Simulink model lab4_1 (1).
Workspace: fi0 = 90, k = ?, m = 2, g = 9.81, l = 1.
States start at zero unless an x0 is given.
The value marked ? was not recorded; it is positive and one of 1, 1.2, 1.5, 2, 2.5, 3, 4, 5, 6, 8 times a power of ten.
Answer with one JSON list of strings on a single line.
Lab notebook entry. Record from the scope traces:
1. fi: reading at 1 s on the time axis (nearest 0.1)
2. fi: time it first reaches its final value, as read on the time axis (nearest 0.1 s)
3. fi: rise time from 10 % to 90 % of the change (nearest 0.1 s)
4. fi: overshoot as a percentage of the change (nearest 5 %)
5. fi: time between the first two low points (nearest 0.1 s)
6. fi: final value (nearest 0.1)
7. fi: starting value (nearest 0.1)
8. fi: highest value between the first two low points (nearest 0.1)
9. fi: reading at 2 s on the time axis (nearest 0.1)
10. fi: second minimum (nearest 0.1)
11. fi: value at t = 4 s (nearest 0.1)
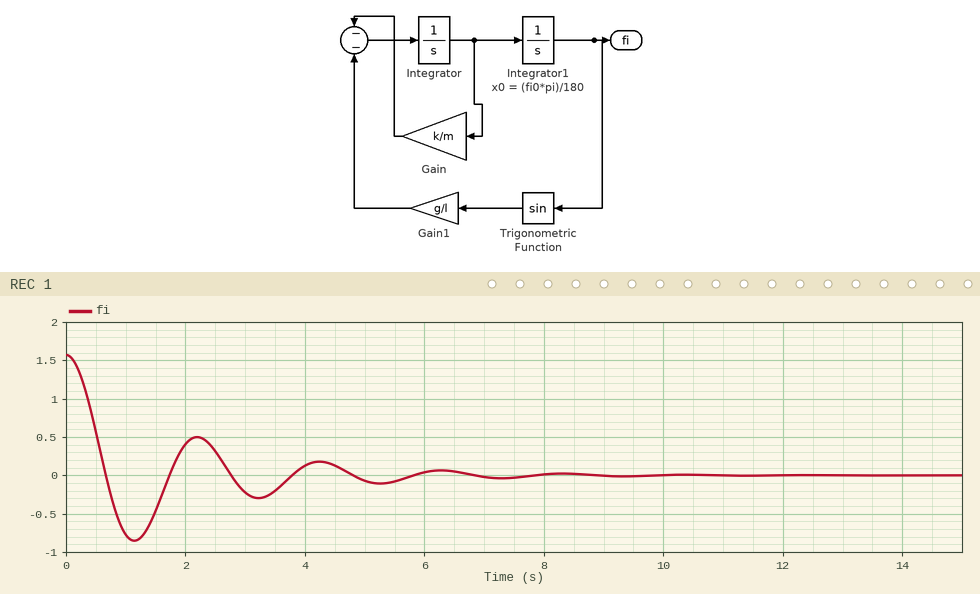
["-0.8", "0.7 s", "0.4 s", "55 %", "2.1 s", "0.0", "1.6", "0.5", "0.4", "-0.3", "0.1"]
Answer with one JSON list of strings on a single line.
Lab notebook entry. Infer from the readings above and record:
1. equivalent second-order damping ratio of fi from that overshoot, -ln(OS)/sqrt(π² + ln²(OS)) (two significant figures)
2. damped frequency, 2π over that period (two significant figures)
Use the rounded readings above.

["0.19", "3.0 rad/s"]
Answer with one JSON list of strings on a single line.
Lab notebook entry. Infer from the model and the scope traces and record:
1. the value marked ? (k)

["2"]
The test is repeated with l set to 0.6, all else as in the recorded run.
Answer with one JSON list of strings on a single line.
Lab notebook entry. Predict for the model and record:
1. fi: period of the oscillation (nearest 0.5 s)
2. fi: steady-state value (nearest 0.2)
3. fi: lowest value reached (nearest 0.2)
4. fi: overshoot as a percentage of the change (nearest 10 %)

["1.5 s", "0.0", "-1.0", "60 %"]
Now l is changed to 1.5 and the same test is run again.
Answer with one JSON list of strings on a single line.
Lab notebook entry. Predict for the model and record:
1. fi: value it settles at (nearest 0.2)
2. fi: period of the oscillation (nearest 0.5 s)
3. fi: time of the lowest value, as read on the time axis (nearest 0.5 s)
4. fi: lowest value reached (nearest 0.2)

["0.0", "2.5 s", "1.5 s", "-0.8"]
